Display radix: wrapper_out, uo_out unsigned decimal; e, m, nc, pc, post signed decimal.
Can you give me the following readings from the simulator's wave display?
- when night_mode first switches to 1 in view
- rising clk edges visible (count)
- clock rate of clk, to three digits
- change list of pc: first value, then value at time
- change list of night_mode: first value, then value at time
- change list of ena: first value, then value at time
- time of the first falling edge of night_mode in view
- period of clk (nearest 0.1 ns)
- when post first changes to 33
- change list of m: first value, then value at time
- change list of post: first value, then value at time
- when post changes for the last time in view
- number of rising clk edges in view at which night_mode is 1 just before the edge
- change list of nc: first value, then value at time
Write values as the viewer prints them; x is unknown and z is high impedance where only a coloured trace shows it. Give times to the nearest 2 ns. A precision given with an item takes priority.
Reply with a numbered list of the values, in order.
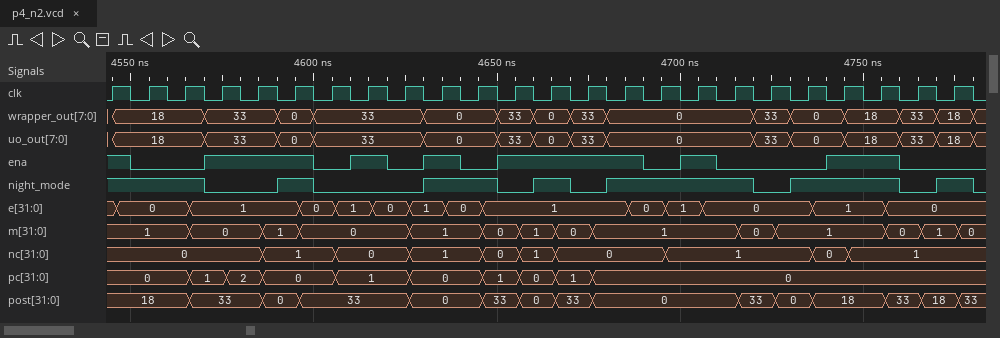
1. 4590 ns
2. 24
3. 100 MHz
4. 0, 1 at 4566 ns, 2 at 4576 ns, 0 at 4586 ns, 1 at 4606 ns, 0 at 4626 ns, 1 at 4646 ns, 0 at 4656 ns, 1 at 4666 ns, 0 at 4676 ns
5. 1, 0 at 4570 ns, 1 at 4590 ns, 0 at 4600 ns, 1 at 4630 ns, 0 at 4650 ns, 1 at 4660 ns, 0 at 4670 ns, 1 at 4680 ns, 0 at 4720 ns, 1 at 4730 ns, 0 at 4760 ns, 1 at 4770 ns, 0 at 4780 ns
6. 1, 0 at 4550 ns, 1 at 4570 ns, 0 at 4600 ns, 1 at 4610 ns, 0 at 4620 ns, 1 at 4630 ns, 0 at 4640 ns, 1 at 4650 ns, 0 at 4690 ns, 1 at 4700 ns, 0 at 4710 ns, 1 at 4740 ns, 0 at 4760 ns
7. 4570 ns
8. 10 ns
9. 4566 ns
10. 1, 0 at 4566 ns, 1 at 4586 ns, 0 at 4596 ns, 1 at 4626 ns, 0 at 4646 ns, 1 at 4656 ns, 0 at 4666 ns, 1 at 4676 ns, 0 at 4716 ns, 1 at 4726 ns, 0 at 4756 ns, 1 at 4766 ns, 0 at 4776 ns
11. 18, 33 at 4566 ns, 0 at 4586 ns, 33 at 4596 ns, 0 at 4626 ns, 33 at 4646 ns, 0 at 4656 ns, 33 at 4666 ns, 0 at 4676 ns, 33 at 4716 ns, 0 at 4726 ns, 18 at 4736 ns, 33 at 4756 ns, 18 at 4766 ns, 33 at 4776 ns
12. 4776 ns
13. 15
14. 0, 1 at 4586 ns, 0 at 4606 ns, 1 at 4626 ns, 0 at 4646 ns, 1 at 4656 ns, 0 at 4666 ns, 1 at 4696 ns, 0 at 4736 ns, 1 at 4746 ns
